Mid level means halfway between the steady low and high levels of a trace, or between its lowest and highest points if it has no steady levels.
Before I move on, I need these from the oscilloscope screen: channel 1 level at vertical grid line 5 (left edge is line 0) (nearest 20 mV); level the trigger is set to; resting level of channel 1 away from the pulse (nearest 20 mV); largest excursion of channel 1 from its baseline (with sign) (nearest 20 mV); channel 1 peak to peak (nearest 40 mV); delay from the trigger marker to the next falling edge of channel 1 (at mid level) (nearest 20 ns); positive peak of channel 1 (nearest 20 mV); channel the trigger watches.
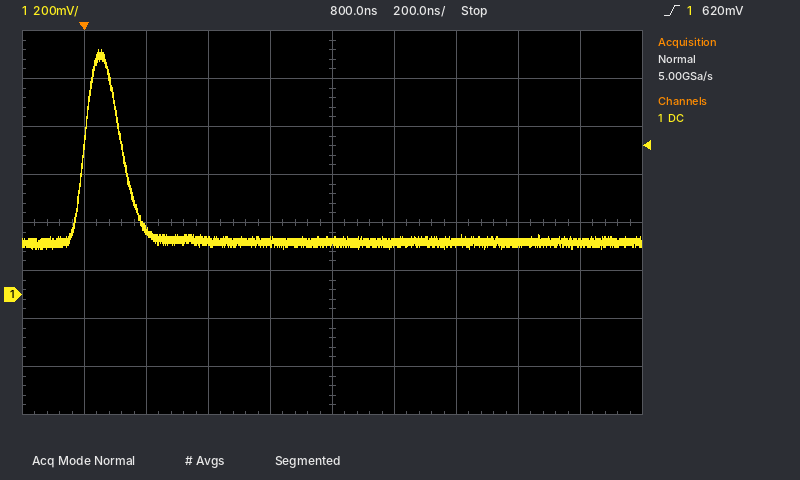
220 mV
620 mV
220 mV
+800 mV
840 mV
120 ns
1.02 V
channel 1
